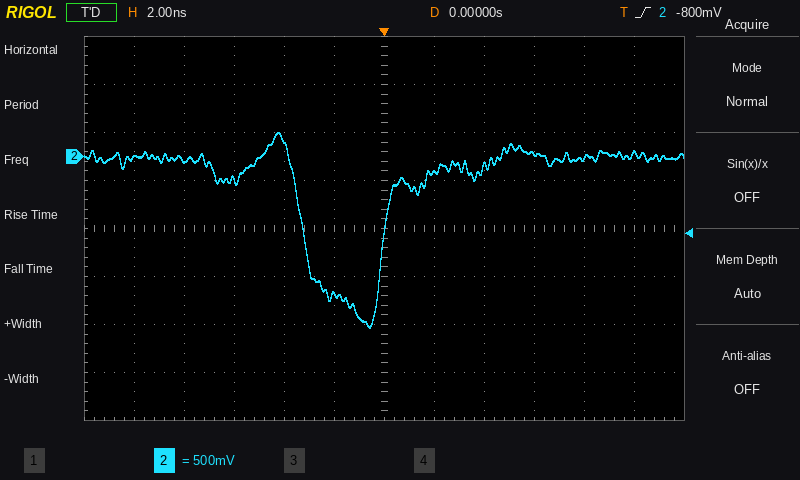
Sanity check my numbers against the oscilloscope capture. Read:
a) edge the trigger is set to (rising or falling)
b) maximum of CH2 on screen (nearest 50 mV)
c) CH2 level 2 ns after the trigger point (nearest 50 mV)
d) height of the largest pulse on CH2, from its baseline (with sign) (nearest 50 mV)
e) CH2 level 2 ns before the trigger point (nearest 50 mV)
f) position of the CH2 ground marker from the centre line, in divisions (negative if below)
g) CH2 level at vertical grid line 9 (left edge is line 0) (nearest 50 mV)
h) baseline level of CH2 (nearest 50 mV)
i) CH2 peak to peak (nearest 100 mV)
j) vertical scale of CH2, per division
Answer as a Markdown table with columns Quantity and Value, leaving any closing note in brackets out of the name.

| Quantity | Value |
|---|---|
| edge the trigger is set to | rising |
| maximum of CH2 on screen | 250 mV |
| CH2 level 2 ns after the trigger point | -150 mV |
| height of the largest pulse on CH2, from its baseline (with sign) | -1.75 V |
| CH2 level 2 ns before the trigger point | -1.45 V |
| position of the CH2 ground marker from the centre line, in divisions | +1.5 div |
| CH2 level at vertical grid line 9 (left edge is line 0) | 50 mV |
| baseline level of CH2 | 0 mV |
| CH2 peak to peak | 2.00 V |
| vertical scale of CH2, per division | 500 mV |
